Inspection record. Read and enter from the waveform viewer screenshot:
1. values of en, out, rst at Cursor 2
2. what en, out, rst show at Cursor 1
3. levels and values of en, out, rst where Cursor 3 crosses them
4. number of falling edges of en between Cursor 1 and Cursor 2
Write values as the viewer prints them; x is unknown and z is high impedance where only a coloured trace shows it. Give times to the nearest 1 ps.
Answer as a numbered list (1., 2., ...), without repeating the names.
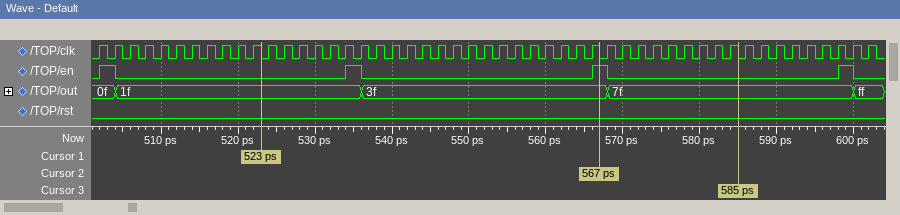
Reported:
1. en=1, out=3f, rst=0
2. en=0, out=1f, rst=0
3. en=0, out=7f, rst=0
4. 1
